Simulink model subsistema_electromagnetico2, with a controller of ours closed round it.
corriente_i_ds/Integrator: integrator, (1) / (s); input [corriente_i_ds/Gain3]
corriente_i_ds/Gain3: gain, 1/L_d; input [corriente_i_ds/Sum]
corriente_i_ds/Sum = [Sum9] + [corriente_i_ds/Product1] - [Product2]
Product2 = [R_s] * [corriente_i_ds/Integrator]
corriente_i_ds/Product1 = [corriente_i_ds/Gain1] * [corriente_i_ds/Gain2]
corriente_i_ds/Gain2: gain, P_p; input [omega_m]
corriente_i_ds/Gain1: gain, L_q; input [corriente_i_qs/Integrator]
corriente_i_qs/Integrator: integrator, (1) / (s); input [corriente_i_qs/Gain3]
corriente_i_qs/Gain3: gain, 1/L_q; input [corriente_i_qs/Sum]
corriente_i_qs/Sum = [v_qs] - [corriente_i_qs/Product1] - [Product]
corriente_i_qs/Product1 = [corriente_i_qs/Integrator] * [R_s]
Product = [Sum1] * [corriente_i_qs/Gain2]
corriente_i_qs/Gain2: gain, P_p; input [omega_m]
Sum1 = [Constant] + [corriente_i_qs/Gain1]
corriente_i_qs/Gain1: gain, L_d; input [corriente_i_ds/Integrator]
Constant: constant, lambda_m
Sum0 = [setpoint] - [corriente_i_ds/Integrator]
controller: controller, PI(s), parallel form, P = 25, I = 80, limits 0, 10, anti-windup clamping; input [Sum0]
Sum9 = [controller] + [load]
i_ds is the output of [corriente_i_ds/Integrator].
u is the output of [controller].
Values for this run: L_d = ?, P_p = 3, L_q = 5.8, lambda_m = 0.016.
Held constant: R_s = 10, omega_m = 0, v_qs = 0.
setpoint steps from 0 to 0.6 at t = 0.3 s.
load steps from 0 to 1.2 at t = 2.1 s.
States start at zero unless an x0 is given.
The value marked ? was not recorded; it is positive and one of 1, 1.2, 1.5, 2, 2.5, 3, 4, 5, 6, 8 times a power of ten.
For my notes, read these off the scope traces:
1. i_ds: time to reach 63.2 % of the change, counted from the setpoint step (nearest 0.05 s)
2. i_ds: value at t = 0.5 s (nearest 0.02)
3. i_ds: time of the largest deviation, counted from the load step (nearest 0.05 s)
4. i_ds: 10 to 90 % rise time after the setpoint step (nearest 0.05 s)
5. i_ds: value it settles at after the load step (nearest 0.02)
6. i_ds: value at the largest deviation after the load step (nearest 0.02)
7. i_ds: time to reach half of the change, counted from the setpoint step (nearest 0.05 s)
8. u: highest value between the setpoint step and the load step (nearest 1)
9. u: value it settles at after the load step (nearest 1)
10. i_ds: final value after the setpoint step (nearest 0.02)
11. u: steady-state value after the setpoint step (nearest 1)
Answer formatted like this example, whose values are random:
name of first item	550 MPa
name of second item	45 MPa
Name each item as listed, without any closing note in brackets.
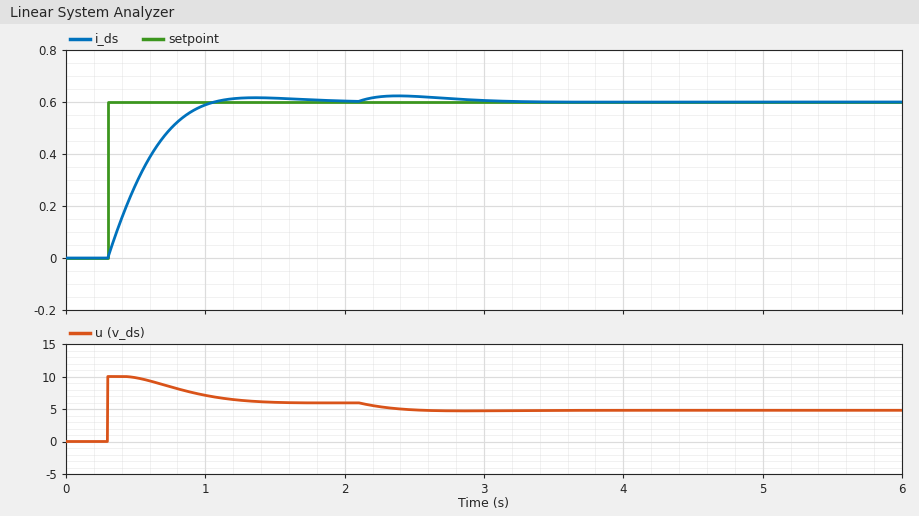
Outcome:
i_ds: time to reach 63.2 % of the change, counted from the setpoint step	0.30 s
i_ds: value at t = 0.5 s	0.28
i_ds: time of the largest deviation, counted from the load step	0.30 s
i_ds: 10 to 90 % rise time after the setpoint step	0.50 s
i_ds: value it settles at after the load step	0.60
i_ds: value at the largest deviation after the load step	0.62
i_ds: time to reach half of the change, counted from the setpoint step	0.20 s
u: highest value between the setpoint step and the load step	10
u: value it settles at after the load step	5
i_ds: final value after the setpoint step	0.60
u: steady-state value after the setpoint step	6
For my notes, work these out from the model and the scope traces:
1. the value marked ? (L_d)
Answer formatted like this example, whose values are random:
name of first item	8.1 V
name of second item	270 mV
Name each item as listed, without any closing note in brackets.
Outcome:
the value marked ?	6
